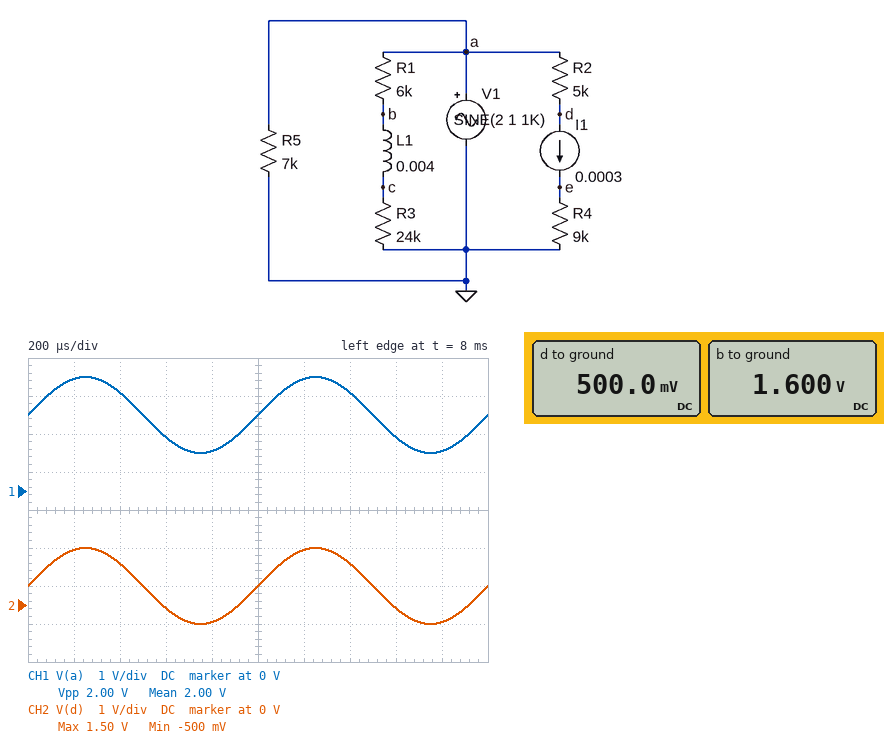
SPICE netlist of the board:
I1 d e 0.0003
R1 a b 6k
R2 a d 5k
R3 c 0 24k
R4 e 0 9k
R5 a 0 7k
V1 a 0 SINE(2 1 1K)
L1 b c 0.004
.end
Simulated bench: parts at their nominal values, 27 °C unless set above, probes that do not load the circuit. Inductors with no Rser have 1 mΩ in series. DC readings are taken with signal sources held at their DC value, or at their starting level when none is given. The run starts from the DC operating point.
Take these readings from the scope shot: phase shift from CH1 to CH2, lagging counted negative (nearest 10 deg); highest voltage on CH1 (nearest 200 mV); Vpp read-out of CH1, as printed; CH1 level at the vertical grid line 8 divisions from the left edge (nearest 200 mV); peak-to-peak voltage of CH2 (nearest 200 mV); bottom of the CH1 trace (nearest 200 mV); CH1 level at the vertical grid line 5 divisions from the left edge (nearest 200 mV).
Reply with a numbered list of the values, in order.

1. 0 deg
2. 3.0 V
3. 2.00 V
4. 1.4 V
5. 2.0 V
6. 1.0 V
7. 2.0 V
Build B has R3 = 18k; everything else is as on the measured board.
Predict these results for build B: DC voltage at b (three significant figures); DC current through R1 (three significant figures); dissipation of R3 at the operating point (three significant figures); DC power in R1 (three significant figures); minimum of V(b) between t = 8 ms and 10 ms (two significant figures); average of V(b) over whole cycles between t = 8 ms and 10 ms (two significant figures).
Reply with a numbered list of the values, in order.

1. 1.50 V
2. 83.3 µA
3. 125 µW
4. 41.7 µW
5. 750 mV
6. 1.5 V
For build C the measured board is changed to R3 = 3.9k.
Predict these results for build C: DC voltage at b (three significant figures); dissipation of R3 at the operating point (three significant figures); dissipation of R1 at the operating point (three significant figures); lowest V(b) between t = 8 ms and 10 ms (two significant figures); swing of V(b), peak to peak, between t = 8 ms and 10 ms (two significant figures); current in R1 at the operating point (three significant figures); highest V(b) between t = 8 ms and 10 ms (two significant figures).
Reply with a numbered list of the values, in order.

1. 788 mV
2. 159 µW
3. 245 µW
4. 390 mV
5. 790 mV
6. 202 µA
7. 1.2 V
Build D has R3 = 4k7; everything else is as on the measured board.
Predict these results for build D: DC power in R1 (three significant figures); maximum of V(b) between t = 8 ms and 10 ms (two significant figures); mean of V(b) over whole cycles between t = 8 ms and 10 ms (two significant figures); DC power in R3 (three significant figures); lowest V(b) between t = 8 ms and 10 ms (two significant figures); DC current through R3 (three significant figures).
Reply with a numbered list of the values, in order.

1. 210 µW
2. 1.3 V
3. 880 mV
4. 164 µW
5. 440 mV
6. 187 µA
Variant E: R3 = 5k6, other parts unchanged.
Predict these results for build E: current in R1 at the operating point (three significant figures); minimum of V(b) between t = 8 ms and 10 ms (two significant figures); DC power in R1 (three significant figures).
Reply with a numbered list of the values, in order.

1. 172 µA
2. 480 mV
3. 178 µW
